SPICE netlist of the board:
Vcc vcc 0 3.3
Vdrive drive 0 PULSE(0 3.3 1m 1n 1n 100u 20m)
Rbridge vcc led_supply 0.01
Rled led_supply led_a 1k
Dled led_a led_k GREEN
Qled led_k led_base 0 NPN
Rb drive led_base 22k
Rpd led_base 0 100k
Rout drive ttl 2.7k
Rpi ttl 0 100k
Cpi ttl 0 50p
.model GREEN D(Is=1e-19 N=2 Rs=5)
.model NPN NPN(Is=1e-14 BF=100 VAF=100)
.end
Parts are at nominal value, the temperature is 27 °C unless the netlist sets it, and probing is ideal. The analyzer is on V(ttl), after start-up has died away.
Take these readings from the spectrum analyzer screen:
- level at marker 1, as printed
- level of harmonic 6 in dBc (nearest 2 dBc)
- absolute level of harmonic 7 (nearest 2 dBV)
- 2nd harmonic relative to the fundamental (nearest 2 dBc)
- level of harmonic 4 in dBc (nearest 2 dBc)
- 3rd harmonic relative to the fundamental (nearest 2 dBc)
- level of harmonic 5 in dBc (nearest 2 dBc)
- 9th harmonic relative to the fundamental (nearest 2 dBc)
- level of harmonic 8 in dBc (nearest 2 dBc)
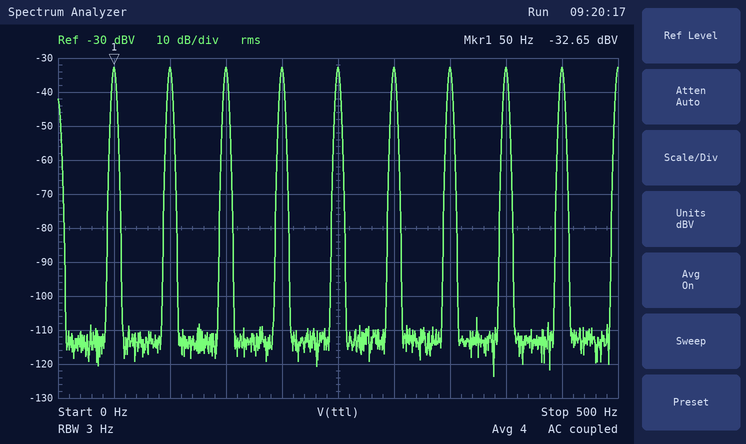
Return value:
-32.65 dBV
0 dBc
-32 dBV
0 dBc
0 dBc
0 dBc
0 dBc
0 dBc
0 dBc
